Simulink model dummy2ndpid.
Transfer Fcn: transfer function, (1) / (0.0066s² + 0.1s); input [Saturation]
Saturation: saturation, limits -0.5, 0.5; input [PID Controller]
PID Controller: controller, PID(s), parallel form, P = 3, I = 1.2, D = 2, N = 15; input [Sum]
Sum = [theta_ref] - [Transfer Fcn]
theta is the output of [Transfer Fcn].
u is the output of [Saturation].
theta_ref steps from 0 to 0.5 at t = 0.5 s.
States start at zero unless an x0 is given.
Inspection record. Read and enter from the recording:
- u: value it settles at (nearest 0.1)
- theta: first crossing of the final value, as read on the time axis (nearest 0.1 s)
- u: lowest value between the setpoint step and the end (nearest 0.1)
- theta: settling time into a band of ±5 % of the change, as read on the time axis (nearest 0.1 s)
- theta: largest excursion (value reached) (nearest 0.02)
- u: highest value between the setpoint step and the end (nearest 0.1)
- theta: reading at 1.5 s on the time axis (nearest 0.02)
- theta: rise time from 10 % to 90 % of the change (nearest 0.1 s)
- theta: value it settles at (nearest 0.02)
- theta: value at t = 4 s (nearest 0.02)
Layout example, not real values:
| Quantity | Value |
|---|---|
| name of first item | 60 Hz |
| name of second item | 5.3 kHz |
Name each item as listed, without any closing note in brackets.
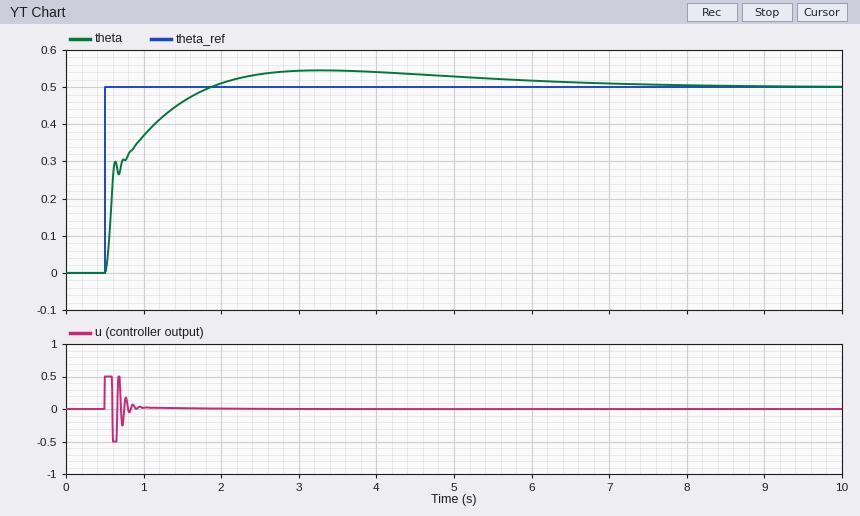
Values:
| Quantity | Value |
|---|---|
| u: value it settles at | 0.0 |
| theta: first crossing of the final value, as read on the time axis | 1.9 s |
| u: lowest value between the setpoint step and the end | -0.5 |
| theta: settling time into a band of ±5 % of the change, as read on the time axis | 5.3 s |
| theta: largest excursion (value reached) | 0.54 |
| u: highest value between the setpoint step and the end | 0.5 |
| theta: reading at 1.5 s on the time axis | 0.46 |
| theta: rise time from 10 % to 90 % of the change | 0.9 s |
| theta: value it settles at | 0.50 |
| theta: value at t = 4 s | 0.54 |
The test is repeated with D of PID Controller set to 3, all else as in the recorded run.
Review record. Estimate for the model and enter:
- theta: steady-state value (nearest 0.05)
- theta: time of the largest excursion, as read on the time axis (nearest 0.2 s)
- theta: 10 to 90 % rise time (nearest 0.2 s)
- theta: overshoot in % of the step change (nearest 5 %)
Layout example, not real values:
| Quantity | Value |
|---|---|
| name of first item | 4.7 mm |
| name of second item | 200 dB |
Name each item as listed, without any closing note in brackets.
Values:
| Quantity | Value |
|---|---|
| theta: steady-state value | 0.50 |
| theta: time of the largest excursion, as read on the time axis | 4.0 s |
| theta: 10 to 90 % rise time | 1.2 s |
| theta: overshoot in % of the step change | 10 % |
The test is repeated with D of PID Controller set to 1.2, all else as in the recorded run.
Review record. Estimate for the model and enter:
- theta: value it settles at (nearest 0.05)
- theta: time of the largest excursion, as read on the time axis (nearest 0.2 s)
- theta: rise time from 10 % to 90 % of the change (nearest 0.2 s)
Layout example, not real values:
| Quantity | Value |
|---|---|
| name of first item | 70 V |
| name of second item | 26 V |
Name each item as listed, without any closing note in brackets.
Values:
| Quantity | Value |
|---|---|
| theta: value it settles at | 0.50 |
| theta: time of the largest excursion, as read on the time axis | 2.6 s |
| theta: rise time from 10 % to 90 % of the change | 0.6 s |
